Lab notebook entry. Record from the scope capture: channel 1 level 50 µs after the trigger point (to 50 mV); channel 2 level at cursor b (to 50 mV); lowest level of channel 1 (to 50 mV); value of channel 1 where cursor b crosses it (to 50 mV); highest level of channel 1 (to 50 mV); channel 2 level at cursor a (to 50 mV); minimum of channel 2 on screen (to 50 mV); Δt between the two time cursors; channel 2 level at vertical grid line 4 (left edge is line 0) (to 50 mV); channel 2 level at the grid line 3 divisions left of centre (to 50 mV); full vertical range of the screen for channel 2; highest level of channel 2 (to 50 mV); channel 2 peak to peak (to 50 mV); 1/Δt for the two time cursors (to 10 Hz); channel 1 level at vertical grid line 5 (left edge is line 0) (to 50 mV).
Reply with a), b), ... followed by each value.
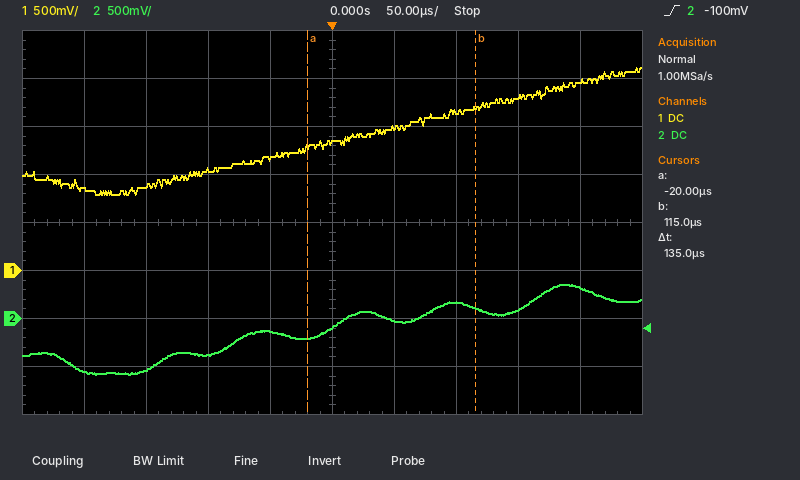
a) 1.50 V
b) 100 mV
c) 800 mV
d) 1.70 V
e) 2.10 V
f) -200 mV
g) -600 mV
h) 135 µs
i) -150 mV
j) -550 mV
k) 4 V
l) 350 mV
m) 950 mV
n) 7.41 kHz
o) 1.35 V
